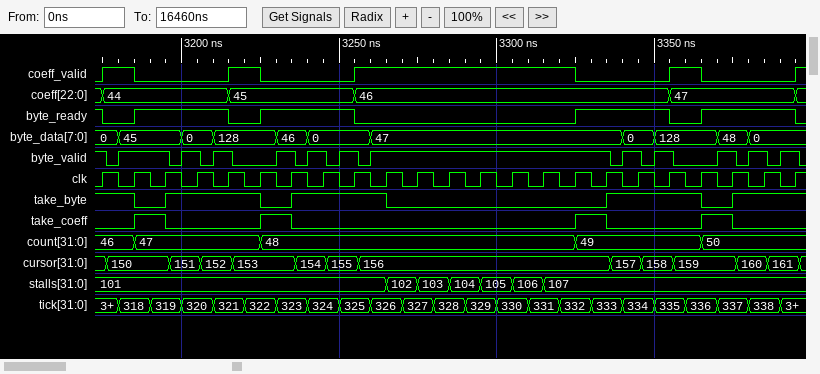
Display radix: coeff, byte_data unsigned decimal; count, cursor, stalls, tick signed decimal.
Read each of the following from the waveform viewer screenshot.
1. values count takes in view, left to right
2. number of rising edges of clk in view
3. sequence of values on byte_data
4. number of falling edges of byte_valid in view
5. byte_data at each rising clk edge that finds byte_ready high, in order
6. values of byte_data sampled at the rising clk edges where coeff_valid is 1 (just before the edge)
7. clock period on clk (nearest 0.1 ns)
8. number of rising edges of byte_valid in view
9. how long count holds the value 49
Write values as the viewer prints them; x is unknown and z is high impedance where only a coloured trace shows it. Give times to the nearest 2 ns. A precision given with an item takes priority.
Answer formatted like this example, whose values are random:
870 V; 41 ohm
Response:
46, 47, 48, 49, 50; 23; 0, 45, 0, 128, 46, 0, 47, 0, 128, 48, 0; 13; 0, 45, 0, 128, 46, 0, 0, 47, 0, 128, 48, 0, 0; 45, 128, 47, 47, 47, 47, 47, 47, 47, 128; 10 ns; 12; 40 ns
